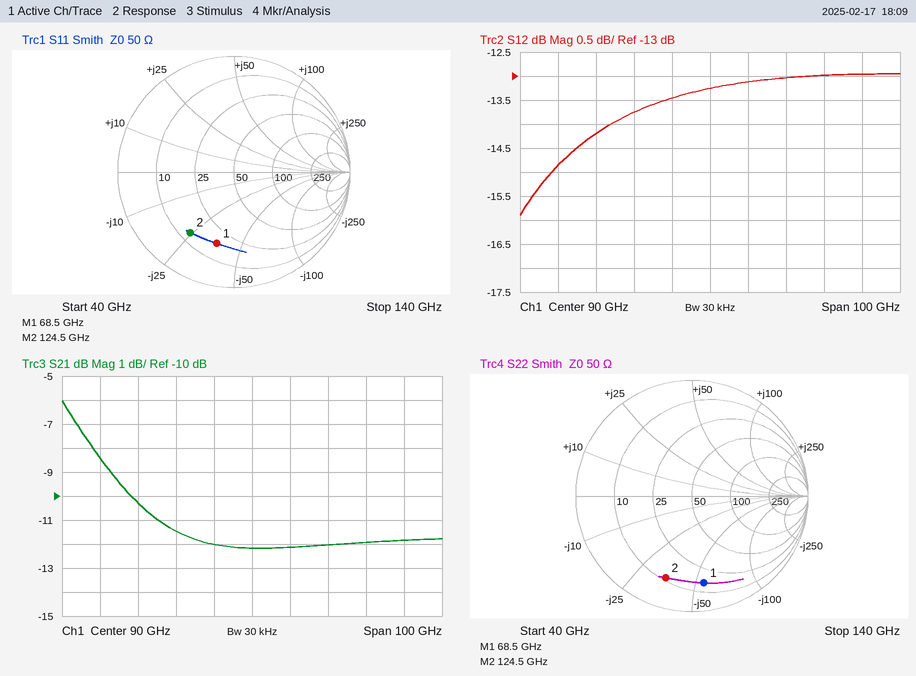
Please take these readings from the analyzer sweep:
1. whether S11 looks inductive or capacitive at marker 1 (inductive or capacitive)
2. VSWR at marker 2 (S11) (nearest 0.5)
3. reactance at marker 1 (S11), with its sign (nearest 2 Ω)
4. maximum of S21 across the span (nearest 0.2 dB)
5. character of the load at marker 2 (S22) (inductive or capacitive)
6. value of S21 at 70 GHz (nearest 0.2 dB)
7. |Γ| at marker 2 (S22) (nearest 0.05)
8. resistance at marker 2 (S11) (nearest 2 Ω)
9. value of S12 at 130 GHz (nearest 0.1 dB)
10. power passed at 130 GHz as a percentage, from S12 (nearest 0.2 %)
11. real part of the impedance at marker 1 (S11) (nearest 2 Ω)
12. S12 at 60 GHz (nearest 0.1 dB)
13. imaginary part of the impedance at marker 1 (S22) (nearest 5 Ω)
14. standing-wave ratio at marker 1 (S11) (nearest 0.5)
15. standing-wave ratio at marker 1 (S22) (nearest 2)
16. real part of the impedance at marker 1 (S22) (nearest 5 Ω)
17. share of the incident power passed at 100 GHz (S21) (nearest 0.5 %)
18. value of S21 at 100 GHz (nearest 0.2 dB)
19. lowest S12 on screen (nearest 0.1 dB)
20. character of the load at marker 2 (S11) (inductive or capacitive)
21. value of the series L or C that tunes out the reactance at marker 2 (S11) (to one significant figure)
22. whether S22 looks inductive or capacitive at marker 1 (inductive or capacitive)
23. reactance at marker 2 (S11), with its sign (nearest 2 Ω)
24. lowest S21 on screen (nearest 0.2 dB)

capacitive
4.5
-36 Ω
-6.0 dB
capacitive
-11.4 dB
0.75
14 Ω
-13.0 dB
5.0 %
18 Ω
-14.2 dB
-55 Ω
4.5
8
15 Ω
6.0 %
-12.2 dB
-15.9 dB
capacitive
30 pH
capacitive
-24 Ω
-12.2 dB
